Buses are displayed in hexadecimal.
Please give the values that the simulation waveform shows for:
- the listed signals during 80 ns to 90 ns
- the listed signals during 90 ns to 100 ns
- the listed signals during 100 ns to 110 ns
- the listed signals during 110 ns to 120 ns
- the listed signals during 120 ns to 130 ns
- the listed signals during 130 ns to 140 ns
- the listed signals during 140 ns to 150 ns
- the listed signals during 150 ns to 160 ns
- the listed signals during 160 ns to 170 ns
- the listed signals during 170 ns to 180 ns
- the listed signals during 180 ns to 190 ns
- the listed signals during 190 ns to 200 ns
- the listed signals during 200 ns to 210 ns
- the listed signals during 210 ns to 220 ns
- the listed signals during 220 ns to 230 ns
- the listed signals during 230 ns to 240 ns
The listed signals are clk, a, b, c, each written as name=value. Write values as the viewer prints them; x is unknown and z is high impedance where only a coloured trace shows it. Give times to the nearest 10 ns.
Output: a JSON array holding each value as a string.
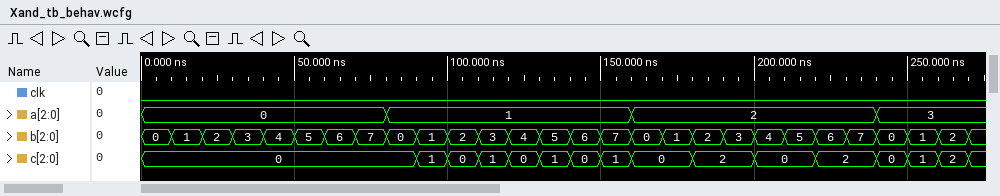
["clk=0, a=1, b=0, c=0", "clk=0, a=1, b=1, c=1", "clk=0, a=1, b=2, c=0", "clk=0, a=1, b=3, c=1", "clk=0, a=1, b=4, c=0", "clk=0, a=1, b=5, c=1", "clk=0, a=1, b=6, c=0", "clk=0, a=1, b=7, c=1", "clk=0, a=2, b=0, c=0", "clk=0, a=2, b=1, c=0", "clk=0, a=2, b=2, c=2", "clk=0, a=2, b=3, c=2", "clk=0, a=2, b=4, c=0", "clk=0, a=2, b=5, c=0", "clk=0, a=2, b=6, c=2", "clk=0, a=2, b=7, c=2"]
